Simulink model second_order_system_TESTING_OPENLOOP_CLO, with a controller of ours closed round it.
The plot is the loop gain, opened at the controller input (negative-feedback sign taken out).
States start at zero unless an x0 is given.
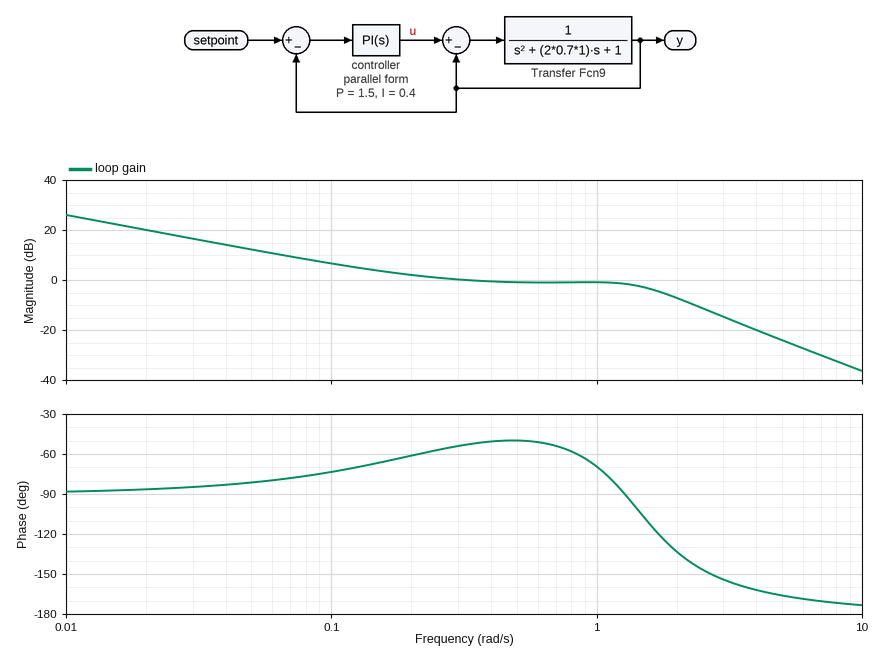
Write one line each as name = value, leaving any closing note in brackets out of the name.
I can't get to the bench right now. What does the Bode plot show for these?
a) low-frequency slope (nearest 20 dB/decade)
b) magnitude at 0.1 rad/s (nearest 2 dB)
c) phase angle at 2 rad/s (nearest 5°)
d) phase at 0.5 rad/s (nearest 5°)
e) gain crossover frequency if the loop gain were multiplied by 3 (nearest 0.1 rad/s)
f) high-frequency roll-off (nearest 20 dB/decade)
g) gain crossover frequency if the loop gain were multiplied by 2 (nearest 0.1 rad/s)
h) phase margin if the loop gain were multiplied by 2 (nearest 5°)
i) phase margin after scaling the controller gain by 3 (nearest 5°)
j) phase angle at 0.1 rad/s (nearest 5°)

low-frequency slope = -20 dB/decade
magnitude at 0.1 rad/s = 6 dB
phase angle at 2 rad/s = -135°
phase at 0.5 rad/s = -50°
gain crossover frequency if the loop gain were multiplied by 3 = 2.3 rad/s
high-frequency roll-off = -40 dB/decade
gain crossover frequency if the loop gain were multiplied by 2 = 1.9 rad/s
phase margin if the loop gain were multiplied by 2 = 50°
phase margin after scaling the controller gain by 3 = 40°
phase angle at 0.1 rad/s = -75°
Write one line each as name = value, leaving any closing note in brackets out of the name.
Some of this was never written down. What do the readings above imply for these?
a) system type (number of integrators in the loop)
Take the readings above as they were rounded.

system type = 1
